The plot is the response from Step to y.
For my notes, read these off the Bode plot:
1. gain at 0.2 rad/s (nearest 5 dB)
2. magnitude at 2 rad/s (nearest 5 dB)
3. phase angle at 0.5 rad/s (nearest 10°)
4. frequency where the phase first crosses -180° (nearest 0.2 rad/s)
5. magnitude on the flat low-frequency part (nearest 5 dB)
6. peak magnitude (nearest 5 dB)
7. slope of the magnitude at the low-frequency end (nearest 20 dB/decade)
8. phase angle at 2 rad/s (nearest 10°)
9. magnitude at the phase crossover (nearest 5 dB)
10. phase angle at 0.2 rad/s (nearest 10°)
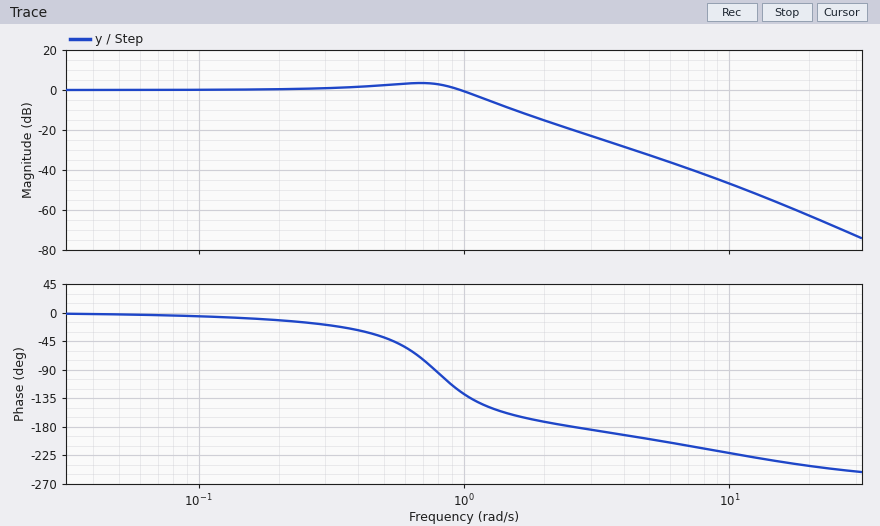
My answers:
0 dB
-15 dB
-40°
2.6 rad/s
0 dB
5 dB
0 dB/decade
-170°
-20 dB
-10°
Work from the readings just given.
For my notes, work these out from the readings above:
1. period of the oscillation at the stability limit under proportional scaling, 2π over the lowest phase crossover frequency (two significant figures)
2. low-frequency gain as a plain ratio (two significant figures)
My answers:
2.4 s
1.0
